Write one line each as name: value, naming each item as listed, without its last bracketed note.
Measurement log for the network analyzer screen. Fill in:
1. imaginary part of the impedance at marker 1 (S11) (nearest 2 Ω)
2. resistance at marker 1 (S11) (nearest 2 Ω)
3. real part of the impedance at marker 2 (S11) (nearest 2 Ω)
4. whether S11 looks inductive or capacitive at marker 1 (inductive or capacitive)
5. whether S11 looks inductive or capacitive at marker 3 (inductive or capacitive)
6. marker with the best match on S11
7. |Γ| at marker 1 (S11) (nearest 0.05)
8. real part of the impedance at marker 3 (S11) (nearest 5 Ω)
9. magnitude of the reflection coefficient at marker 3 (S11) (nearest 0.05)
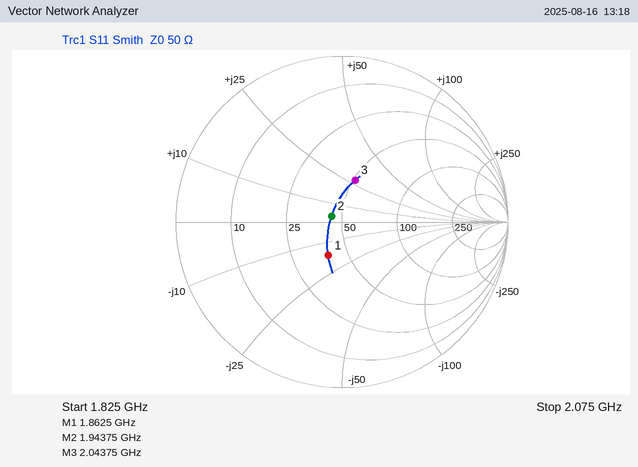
imaginary part of the impedance at marker 1 (S11): -16 Ω
resistance at marker 1 (S11): 40 Ω
real part of the impedance at marker 2 (S11): 44 Ω
whether S11 looks inductive or capacitive at marker 1: capacitive
whether S11 looks inductive or capacitive at marker 3: inductive
marker with the best match on S11: marker 2
|Γ| at marker 1 (S11): 0.20
real part of the impedance at marker 3 (S11): 50 Ω
magnitude of the reflection coefficient at marker 3 (S11): 0.25
